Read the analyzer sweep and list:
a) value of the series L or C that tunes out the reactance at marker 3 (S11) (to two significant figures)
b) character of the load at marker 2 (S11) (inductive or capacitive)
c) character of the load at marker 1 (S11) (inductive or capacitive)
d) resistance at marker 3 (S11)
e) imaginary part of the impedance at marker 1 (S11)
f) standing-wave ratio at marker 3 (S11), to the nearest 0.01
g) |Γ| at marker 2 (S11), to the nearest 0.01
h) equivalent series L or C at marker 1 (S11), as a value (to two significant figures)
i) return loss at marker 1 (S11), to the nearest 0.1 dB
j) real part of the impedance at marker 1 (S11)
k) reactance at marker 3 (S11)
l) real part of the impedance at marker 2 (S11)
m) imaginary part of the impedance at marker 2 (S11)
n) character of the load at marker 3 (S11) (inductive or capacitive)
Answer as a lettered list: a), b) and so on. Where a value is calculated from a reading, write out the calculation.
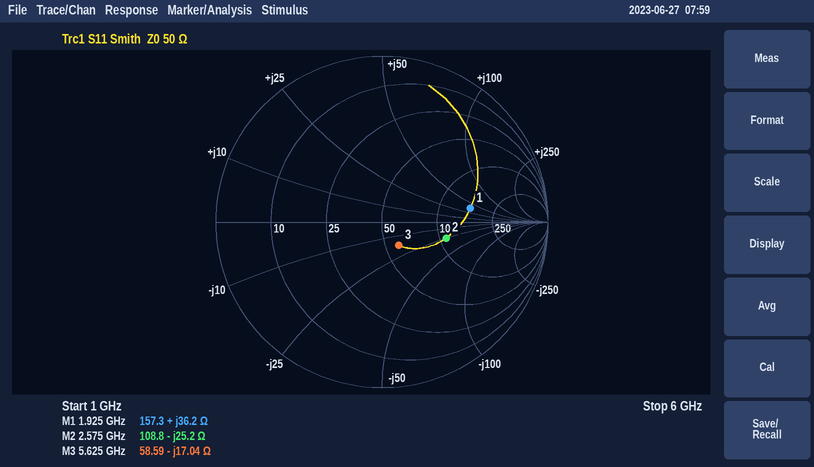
a) L = 17.04 Ω/(2π × 5.625 GHz) ≈ 482 pH, so 480 pH to two significant figures
b) capacitive
c) inductive
d) 58.59 Ω
e) +36.2 Ω
f) 1.42
g) 0.40
h) L = 36.2 Ω/(2π × 1.925 GHz) ≈ 3.0 nH
i) 5.4 dB
j) 157.3 Ω
k) -17.04 Ω
l) 108.8 Ω
m) -25.2 Ω
n) capacitive
